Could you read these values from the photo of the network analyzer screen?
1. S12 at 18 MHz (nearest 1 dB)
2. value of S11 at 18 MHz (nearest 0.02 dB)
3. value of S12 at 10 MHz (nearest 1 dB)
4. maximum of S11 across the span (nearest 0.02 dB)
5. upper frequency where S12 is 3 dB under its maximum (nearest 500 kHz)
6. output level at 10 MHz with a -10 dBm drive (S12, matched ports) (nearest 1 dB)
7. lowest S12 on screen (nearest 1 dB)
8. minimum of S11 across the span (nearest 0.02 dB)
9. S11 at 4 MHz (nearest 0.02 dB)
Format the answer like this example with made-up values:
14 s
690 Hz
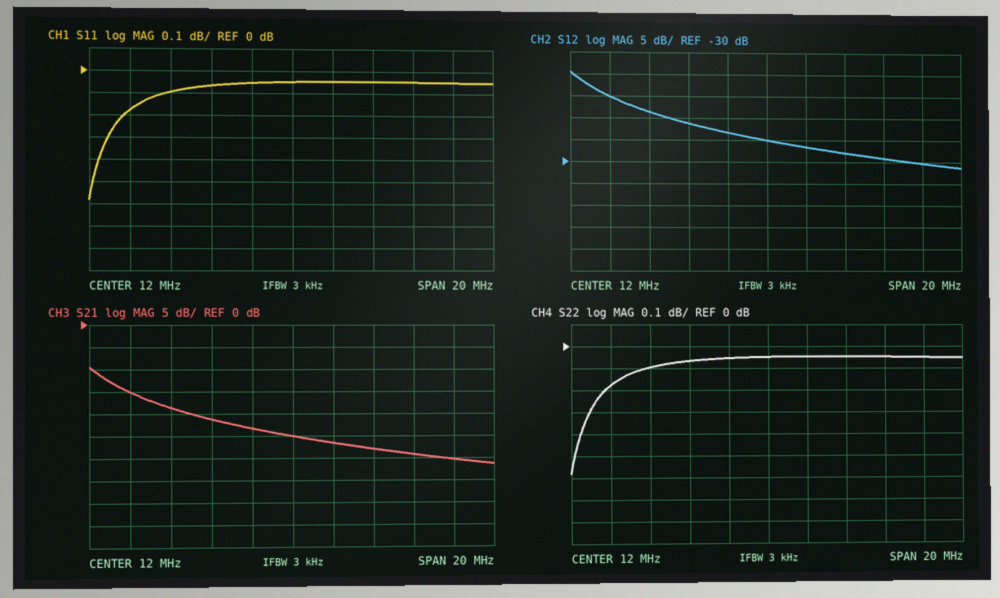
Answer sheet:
-29 dB
-0.04 dB
-23 dB
-0.04 dB
3.0 MHz
-33 dBm
-31 dB
-0.58 dB
-0.18 dB
